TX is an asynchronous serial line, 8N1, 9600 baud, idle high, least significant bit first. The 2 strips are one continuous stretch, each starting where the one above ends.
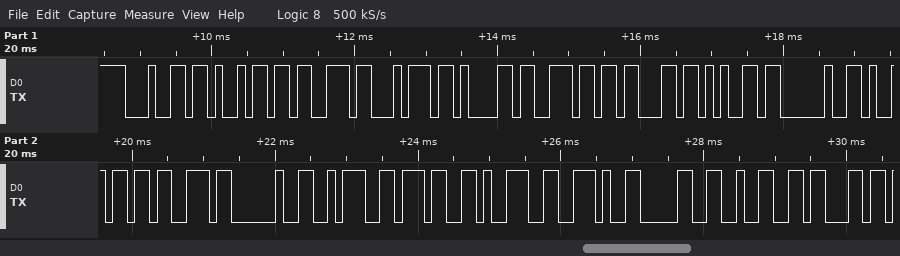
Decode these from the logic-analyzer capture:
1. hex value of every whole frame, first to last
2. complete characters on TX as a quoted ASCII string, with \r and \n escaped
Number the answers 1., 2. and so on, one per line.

1. 64 69 73 74 61 6E 63 65 20 69 73 20 3A 37 39 2E 30 32 63
2. "distance is :79.02c"
